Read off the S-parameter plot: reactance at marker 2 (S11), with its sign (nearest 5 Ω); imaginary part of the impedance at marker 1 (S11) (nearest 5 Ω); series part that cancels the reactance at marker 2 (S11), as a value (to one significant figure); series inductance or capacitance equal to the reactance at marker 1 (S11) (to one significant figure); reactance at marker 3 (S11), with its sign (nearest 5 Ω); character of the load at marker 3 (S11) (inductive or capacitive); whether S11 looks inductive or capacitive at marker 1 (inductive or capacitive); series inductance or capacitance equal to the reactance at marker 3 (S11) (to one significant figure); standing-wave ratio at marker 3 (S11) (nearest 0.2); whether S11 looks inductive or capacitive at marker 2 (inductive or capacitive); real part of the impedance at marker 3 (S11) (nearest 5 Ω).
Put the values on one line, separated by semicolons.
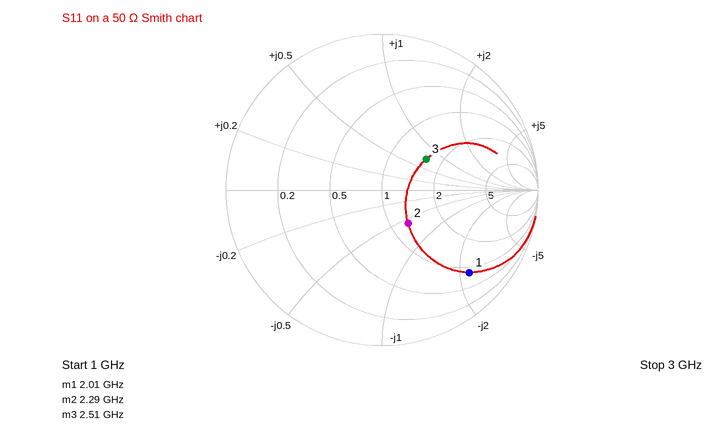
-30 Ω; -110 Ω; 2 nH; 700 fF; +35 Ω; inductive; capacitive; 2 nH; 2.0; capacitive; 80 Ω
